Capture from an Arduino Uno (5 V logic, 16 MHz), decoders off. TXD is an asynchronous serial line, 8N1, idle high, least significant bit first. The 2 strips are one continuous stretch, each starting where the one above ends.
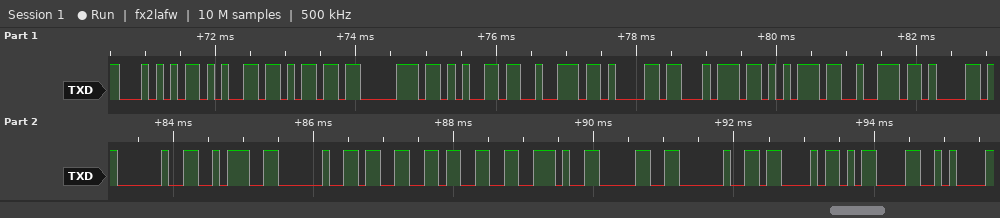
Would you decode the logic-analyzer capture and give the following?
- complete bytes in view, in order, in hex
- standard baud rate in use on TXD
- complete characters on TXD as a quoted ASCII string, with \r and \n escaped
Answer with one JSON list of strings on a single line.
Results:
["54 65 6D 70 65 72 61 74 75 72 61 20 3A 20 33 33 2E 30 20 43 0D 0A", "9600 baud", "\"Temperatura : 33.0 C\\r\\n\""]
